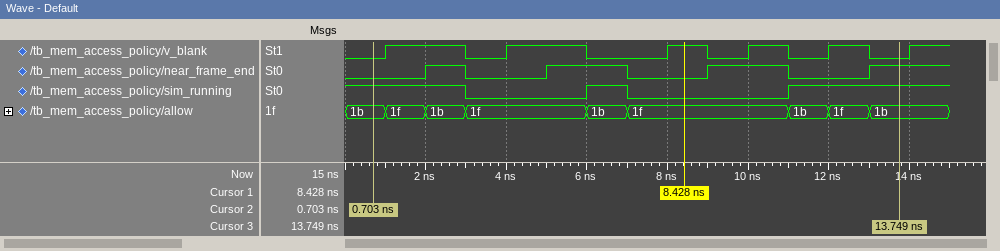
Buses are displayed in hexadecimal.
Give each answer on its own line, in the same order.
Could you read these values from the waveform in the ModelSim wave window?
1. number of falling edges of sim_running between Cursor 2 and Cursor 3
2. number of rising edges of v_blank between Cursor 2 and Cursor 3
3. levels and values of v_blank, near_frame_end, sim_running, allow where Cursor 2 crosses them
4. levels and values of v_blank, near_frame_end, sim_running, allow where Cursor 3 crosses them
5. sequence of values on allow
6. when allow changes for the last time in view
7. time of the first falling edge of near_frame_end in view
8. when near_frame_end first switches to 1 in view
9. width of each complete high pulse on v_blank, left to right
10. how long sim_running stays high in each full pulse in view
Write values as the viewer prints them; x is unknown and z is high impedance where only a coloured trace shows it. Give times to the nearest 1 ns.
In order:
2
5
v_blank=0, near_frame_end=0, sim_running=1, allow=1b
v_blank=0, near_frame_end=1, sim_running=1, allow=1b
1b, 1f, 1b, 1f, 1b, 1f, 1b, 1f, 1b
13 ns
3 ns
2 ns
2 ns, 2 ns, 1 ns, 1 ns, 1 ns
1 ns
